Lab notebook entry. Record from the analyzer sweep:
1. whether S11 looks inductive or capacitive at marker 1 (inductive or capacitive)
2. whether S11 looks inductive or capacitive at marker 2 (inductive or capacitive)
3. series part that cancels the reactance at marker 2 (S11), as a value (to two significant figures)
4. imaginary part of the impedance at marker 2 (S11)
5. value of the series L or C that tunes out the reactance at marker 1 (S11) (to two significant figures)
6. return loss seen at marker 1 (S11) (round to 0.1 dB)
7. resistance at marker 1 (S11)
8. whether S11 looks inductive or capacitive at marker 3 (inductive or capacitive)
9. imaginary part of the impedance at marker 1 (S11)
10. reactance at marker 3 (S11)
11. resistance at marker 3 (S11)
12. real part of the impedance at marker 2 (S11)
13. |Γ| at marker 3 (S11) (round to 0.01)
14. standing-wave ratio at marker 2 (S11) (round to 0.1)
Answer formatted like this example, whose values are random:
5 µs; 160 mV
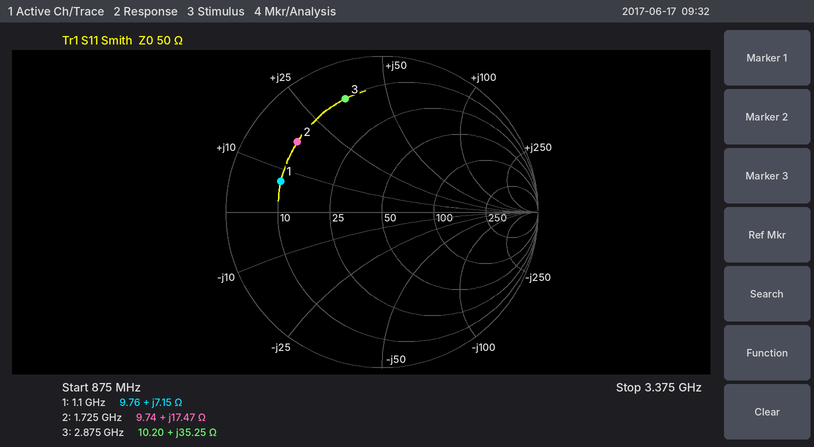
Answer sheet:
inductive; inductive; 5.3 pF; +17.47 Ω; 20 pF; 3.4 dB; 9.76 Ω; inductive; +7.15 Ω; +35.25 Ω; 10.20 Ω; 9.74 Ω; 0.76; 5.8
